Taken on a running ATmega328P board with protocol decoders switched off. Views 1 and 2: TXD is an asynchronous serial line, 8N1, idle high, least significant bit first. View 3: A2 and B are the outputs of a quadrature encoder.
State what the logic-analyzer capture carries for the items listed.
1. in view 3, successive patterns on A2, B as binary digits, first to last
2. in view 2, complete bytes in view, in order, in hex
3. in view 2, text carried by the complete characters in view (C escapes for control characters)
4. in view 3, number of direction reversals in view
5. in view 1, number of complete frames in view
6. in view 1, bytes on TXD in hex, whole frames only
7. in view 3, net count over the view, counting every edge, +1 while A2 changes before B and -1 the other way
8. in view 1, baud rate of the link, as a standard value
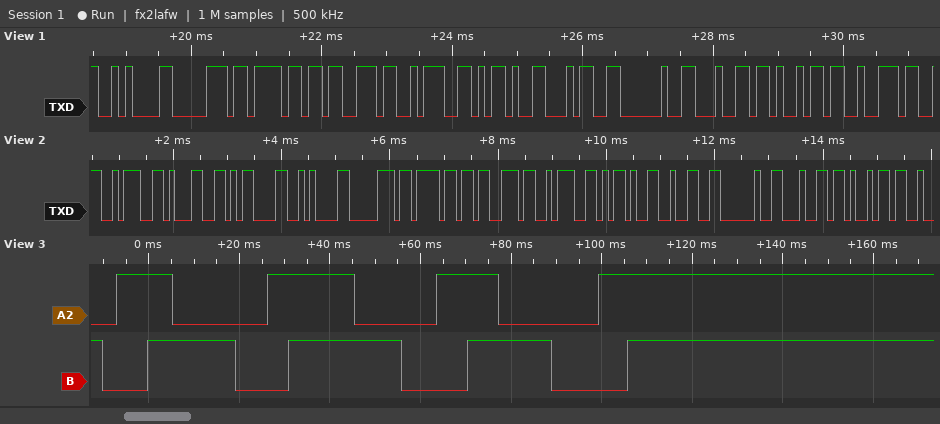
01 00 10 11 01 00 10 11 01 00 10 11 01 00 10 11
3A 31 0D 0A 70 6F 73 3A 2D 32 20 64 69
":1\r\npos:-2 di"
0
11
0A 70 6F 73 3A 2D 34 20 64 69 72
+15
9600 baud
